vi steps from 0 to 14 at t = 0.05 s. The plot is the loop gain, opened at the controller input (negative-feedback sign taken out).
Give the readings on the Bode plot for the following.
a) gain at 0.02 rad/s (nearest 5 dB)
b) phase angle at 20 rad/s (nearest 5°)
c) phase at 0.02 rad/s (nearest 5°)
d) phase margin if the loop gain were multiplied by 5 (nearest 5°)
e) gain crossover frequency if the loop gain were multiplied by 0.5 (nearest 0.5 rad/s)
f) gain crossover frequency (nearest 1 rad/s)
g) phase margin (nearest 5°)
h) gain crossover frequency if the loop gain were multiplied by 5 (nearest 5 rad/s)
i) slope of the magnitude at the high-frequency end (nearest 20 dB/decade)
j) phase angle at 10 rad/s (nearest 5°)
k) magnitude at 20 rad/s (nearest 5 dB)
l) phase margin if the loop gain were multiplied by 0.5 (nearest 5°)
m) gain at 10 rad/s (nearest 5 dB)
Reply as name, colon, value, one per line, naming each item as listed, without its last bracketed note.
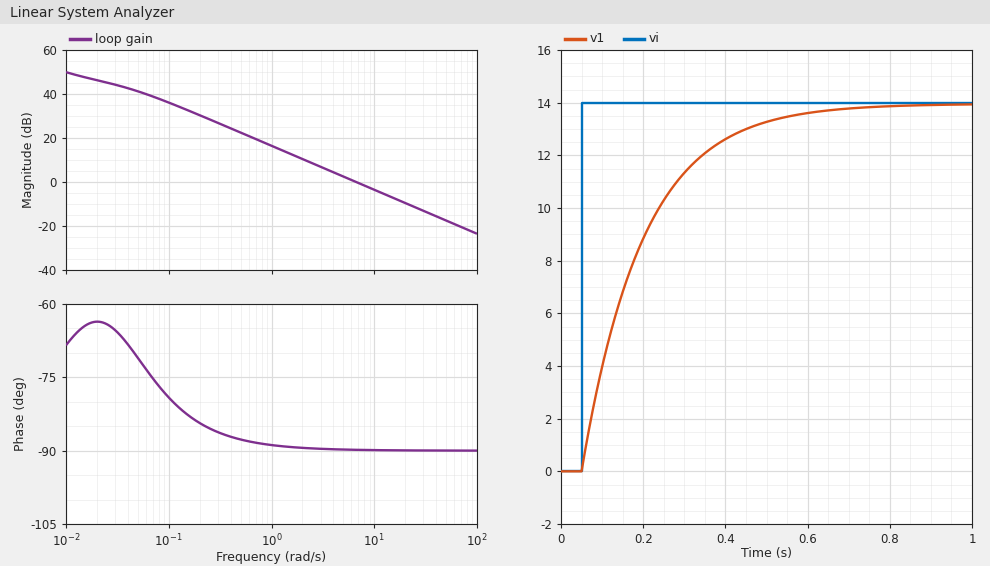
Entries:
gain at 0.02 rad/s: 45 dB
phase angle at 20 rad/s: -90°
phase at 0.02 rad/s: -65°
phase margin if the loop gain were multiplied by 5: 90°
gain crossover frequency if the loop gain were multiplied by 0.5: 3.5 rad/s
gain crossover frequency: 7 rad/s
phase margin: 90°
gain crossover frequency if the loop gain were multiplied by 5: 35 rad/s
slope of the magnitude at the high-frequency end: -20 dB/decade
phase angle at 10 rad/s: -90°
magnitude at 20 rad/s: -10 dB
phase margin if the loop gain were multiplied by 0.5: 90°
gain at 10 rad/s: -5 dB
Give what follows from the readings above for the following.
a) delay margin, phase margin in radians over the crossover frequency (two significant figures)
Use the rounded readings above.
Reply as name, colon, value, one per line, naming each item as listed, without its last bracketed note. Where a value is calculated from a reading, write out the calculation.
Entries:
delay margin, phase margin in radians over the crossover frequency: 90 × π / 180 / 7 = 0.22 s
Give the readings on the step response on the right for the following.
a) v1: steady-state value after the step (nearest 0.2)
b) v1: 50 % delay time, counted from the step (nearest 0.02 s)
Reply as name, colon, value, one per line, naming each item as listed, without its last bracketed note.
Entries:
v1: steady-state value after the step: 14.0
v1: 50 % delay time, counted from the step: 0.10 s
